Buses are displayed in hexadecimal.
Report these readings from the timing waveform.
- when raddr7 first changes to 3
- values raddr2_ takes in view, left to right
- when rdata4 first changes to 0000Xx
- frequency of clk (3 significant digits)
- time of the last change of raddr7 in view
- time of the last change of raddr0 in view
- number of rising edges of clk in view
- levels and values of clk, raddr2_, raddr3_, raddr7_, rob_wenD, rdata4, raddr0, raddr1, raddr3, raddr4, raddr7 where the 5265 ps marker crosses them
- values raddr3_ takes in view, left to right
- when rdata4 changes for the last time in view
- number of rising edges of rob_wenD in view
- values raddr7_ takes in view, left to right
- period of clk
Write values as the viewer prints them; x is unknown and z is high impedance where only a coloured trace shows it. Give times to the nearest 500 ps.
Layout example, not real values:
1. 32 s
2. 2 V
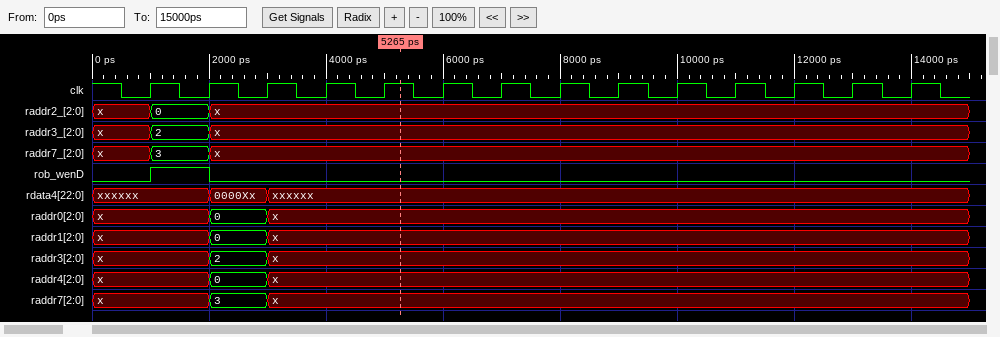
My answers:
1. 2000 ps
2. x, 0, x
3. 2000 ps
4. 1.00 GHz
5. 3000 ps
6. 3000 ps
7. 14
8. clk=1, raddr2_=x, raddr3_=x, raddr7_=x, rob_wenD=0, rdata4=xxxxxx, raddr0=x, raddr1=x, raddr3=x, raddr4=x, raddr7=x
9. x, 2, x
10. 3000 ps
11. 1
12. x, 3, x
13. 1000 ps
